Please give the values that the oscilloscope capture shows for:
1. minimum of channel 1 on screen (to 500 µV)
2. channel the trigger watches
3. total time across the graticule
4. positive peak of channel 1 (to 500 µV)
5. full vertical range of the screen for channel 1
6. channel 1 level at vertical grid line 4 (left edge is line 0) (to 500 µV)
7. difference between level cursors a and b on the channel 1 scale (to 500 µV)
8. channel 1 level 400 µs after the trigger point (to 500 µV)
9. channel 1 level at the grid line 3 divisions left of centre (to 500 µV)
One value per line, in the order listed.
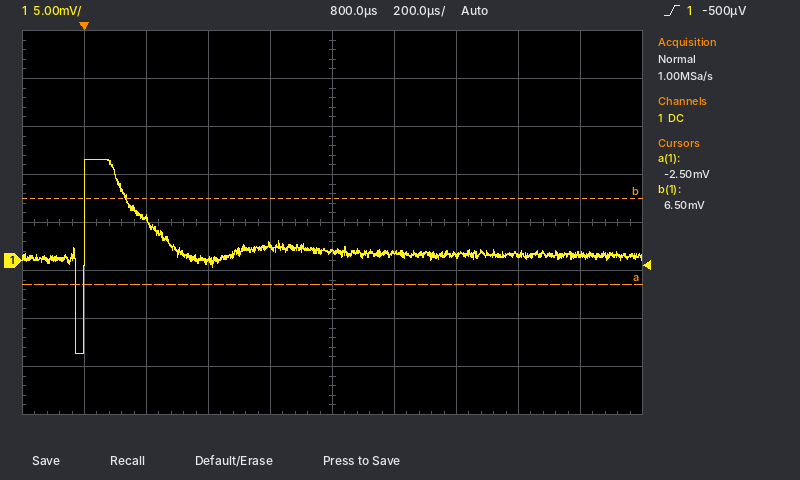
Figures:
-9.5 mV
channel 1
2 ms
10.5 mV
40 mV
1.5 mV
9.0 mV
0.0 mV
4.5 mV
